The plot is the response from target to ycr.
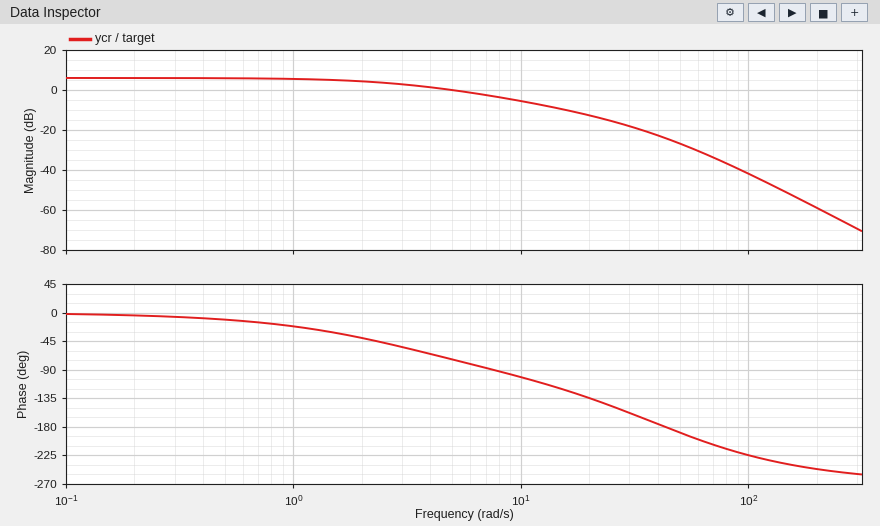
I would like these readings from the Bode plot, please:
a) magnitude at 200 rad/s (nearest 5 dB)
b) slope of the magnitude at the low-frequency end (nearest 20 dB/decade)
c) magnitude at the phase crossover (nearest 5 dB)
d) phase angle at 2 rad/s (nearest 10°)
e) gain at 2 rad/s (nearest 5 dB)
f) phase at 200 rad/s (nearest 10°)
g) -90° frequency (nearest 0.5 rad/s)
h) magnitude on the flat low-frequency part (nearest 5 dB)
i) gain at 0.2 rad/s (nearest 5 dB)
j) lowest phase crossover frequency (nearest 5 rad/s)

-60 dB
0 dB/decade
-25 dB
-40°
5 dB
-250°
7.5 rad/s
5 dB
5 dB
45 rad/s
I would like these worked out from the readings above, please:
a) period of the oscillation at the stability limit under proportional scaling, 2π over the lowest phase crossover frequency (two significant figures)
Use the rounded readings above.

0.14 s
